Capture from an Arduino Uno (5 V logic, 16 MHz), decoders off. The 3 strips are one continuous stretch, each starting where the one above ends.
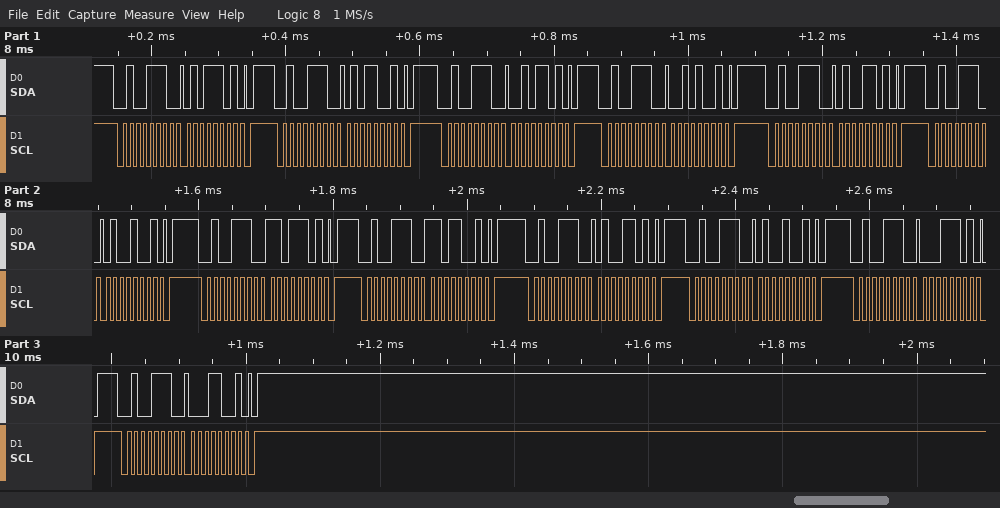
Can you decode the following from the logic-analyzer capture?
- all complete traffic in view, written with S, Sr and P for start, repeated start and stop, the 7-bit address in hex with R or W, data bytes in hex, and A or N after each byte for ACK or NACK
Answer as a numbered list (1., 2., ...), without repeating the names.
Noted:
1. S 27W A 5D A P S 27W A 59 A P S 27W A 2D A P S 27W A 29 A P S 27W A 4D A P S 27W A 49 A P S 27W A DD A P S 27W A D9 A P S 27W A 4D A P S 27W A 49 A P S 27W A 1D A P S 27W A 19 A P
